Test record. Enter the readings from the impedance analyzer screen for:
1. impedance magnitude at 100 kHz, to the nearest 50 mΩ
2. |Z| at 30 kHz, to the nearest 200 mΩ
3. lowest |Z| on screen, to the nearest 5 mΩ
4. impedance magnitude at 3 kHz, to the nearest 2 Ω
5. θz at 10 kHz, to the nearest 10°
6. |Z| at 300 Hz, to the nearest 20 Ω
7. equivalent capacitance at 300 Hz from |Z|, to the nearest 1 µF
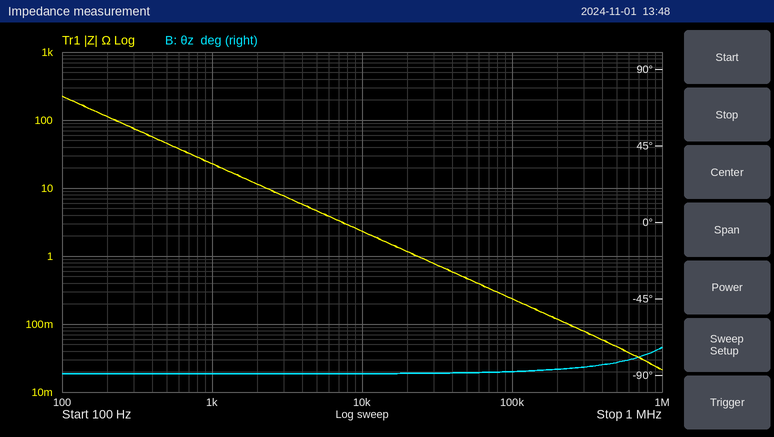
250 mΩ
800 mΩ
20 mΩ
8 Ω
-90°
80 Ω
7 µF
